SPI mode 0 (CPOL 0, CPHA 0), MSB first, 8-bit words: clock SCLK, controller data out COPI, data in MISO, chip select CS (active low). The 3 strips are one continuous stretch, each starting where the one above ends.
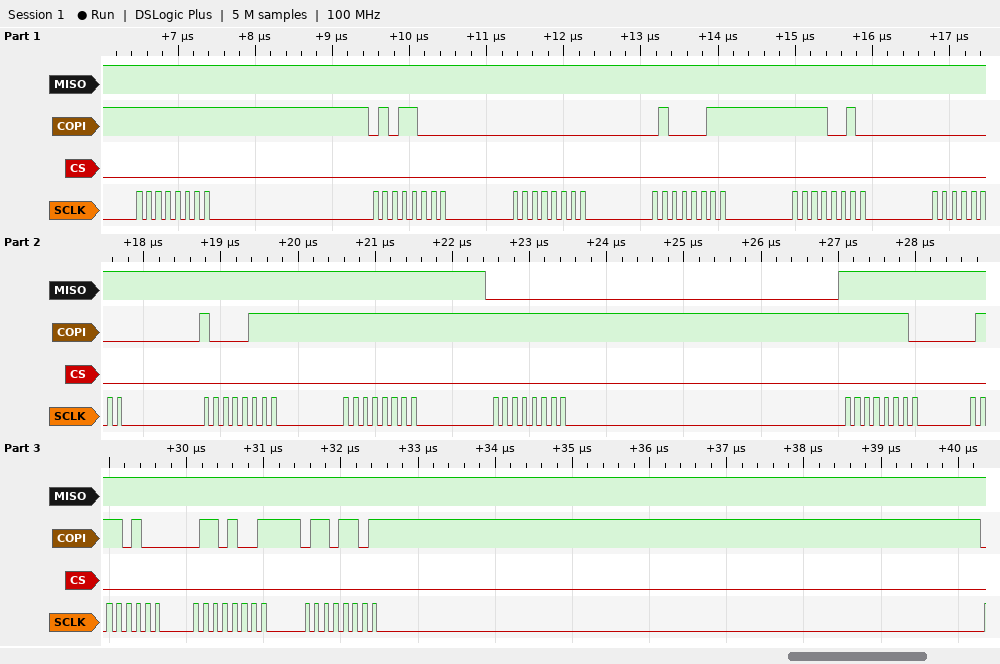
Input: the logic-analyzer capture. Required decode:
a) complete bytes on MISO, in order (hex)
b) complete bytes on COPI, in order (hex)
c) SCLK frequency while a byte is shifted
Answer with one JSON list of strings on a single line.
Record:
["FF FF FF FF FF FF FF FF 00 FF FF FF FF", "FF 58 00 43 F2 00 87 FF FF FE 74 69 6D", "8 MHz"]
